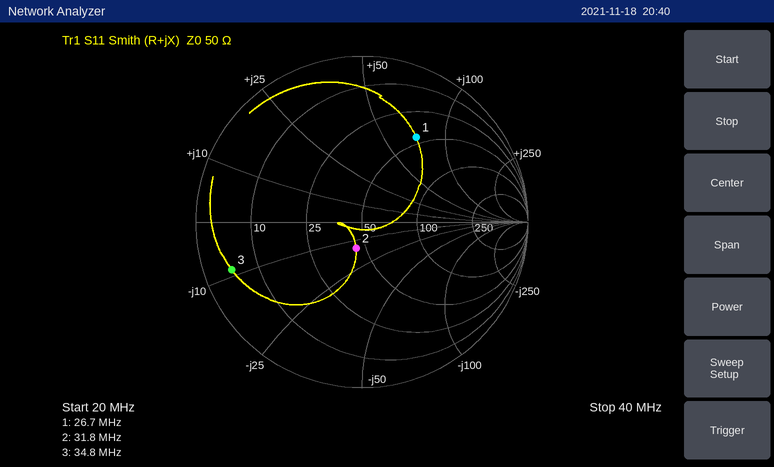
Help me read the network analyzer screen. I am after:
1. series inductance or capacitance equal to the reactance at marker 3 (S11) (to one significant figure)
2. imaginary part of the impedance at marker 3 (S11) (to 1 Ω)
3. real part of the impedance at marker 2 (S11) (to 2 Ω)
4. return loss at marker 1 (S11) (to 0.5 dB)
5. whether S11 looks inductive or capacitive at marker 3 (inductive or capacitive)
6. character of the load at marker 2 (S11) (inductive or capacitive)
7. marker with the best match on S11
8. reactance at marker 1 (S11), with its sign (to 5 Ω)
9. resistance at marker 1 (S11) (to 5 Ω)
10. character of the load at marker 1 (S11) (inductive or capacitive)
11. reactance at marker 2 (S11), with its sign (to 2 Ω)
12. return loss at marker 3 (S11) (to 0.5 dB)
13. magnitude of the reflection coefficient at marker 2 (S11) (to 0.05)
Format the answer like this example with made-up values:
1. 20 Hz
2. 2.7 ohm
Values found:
1. 500 pF
2. -9 Ω
3. 44 Ω
4. 4.5 dB
5. capacitive
6. capacitive
7. marker 2
8. +70 Ω
9. 45 Ω
10. inductive
11. -14 Ω
12. 1.5 dB
13. 0.15
